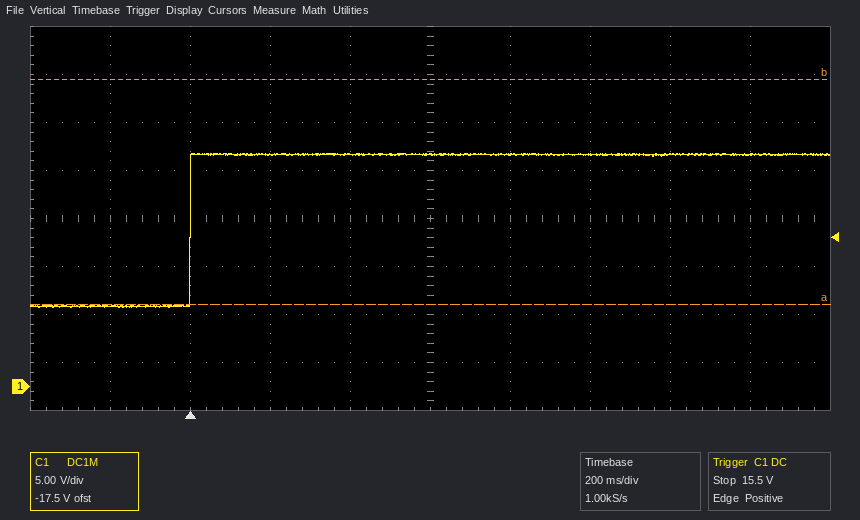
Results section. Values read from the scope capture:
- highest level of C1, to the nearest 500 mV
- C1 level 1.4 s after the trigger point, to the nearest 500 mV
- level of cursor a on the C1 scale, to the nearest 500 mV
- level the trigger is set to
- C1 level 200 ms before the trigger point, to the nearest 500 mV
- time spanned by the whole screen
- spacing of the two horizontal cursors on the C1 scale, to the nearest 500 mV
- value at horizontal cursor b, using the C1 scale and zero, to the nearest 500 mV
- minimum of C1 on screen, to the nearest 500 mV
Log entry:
24.5 V
24.0 V
8.5 V
15.5 V
8.5 V
2 s
23.5 V
32.0 V
8.0 V
